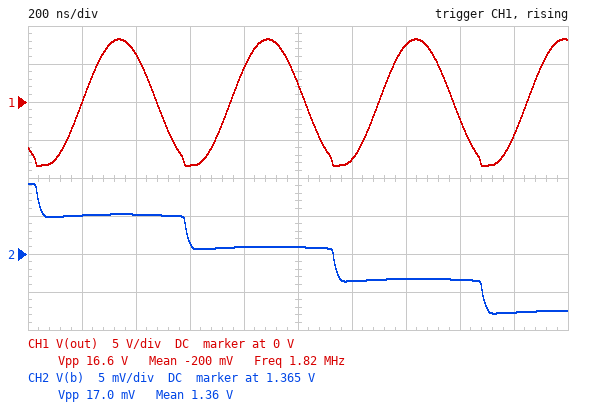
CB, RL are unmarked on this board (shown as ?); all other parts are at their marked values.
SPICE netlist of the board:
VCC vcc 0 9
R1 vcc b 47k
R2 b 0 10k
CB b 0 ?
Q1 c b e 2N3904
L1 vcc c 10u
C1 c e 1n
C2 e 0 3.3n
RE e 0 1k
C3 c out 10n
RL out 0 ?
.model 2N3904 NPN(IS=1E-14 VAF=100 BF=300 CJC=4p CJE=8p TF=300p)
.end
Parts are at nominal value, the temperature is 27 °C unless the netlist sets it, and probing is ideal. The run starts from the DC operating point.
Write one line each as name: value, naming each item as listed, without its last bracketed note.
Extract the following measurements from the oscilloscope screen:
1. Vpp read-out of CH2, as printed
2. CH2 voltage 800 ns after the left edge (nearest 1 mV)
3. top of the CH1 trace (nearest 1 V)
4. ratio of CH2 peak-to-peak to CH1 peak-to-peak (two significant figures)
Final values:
Vpp read-out of CH2, as printed: 17.0 mV
CH2 voltage 800 ns after the left edge: 1.366 V
top of the CH1 trace: 8 V
ratio of CH2 peak-to-peak to CH1 peak-to-peak: 0.0010
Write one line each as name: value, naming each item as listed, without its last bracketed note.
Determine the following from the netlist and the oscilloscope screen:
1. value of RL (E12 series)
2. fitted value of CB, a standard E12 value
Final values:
value of RL: 27 kΩ
fitted value of CB, a standard E12 value: 180 nF
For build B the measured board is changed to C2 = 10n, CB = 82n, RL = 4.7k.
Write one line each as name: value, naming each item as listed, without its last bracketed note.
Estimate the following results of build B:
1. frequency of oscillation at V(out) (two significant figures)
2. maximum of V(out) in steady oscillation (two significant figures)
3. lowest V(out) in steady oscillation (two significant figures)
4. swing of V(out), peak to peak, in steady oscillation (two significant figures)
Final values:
frequency of oscillation at V(out): 1.7 MHz
maximum of V(out) in steady oscillation: 8.1 V
lowest V(out) in steady oscillation: -8.3 V
swing of V(out), peak to peak, in steady oscillation: 16 V
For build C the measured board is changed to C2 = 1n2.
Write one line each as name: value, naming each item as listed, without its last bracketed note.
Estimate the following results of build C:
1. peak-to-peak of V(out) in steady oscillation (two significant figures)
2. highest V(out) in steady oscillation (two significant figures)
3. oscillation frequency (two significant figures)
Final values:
peak-to-peak of V(out) in steady oscillation: 16 V
highest V(out) in steady oscillation: 7.9 V
oscillation frequency: 2.2 MHz
